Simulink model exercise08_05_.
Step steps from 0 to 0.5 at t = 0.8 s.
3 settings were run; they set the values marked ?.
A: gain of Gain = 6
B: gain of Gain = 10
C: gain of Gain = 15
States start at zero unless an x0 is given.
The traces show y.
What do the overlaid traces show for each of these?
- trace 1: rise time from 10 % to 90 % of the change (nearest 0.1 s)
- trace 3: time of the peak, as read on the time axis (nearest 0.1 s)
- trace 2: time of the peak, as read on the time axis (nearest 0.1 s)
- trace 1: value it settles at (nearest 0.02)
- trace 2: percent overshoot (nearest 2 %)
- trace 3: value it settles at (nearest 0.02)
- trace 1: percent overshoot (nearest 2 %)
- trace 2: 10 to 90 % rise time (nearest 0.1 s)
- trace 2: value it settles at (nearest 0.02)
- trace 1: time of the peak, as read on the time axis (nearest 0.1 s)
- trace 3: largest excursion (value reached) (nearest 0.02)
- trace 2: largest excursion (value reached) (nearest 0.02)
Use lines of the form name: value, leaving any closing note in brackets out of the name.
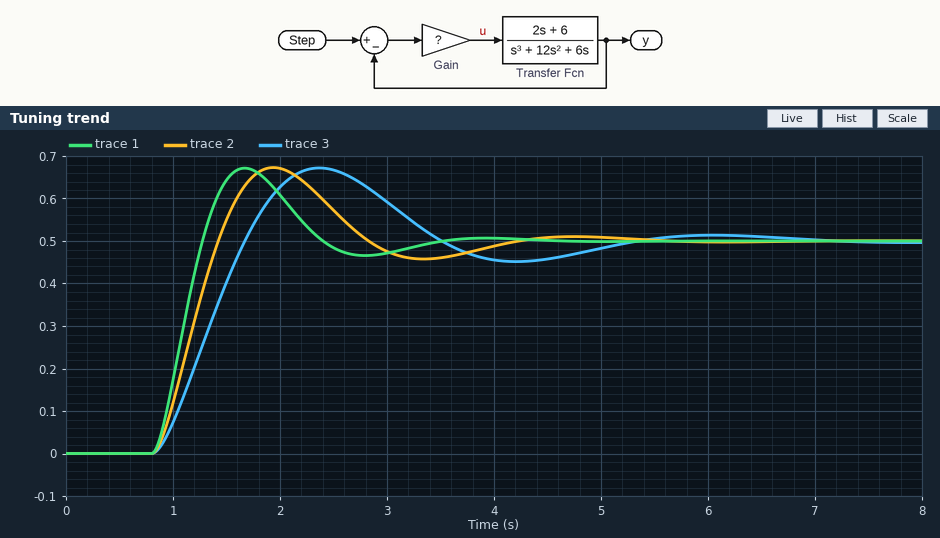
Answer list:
trace 1: rise time from 10 % to 90 % of the change: 0.3 s
trace 3: time of the peak, as read on the time axis: 2.4 s
trace 2: time of the peak, as read on the time axis: 1.9 s
trace 1: value it settles at: 0.50
trace 2: percent overshoot: 34 %
trace 3: value it settles at: 0.50
trace 1: percent overshoot: 34 %
trace 2: 10 to 90 % rise time: 0.4 s
trace 2: value it settles at: 0.50
trace 1: time of the peak, as read on the time axis: 1.7 s
trace 3: largest excursion (value reached): 0.68
trace 2: largest excursion (value reached): 0.68
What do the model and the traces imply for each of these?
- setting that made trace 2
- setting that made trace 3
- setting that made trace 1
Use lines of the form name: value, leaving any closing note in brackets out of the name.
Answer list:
setting that made trace 2: B
setting that made trace 3: A
setting that made trace 1: C
